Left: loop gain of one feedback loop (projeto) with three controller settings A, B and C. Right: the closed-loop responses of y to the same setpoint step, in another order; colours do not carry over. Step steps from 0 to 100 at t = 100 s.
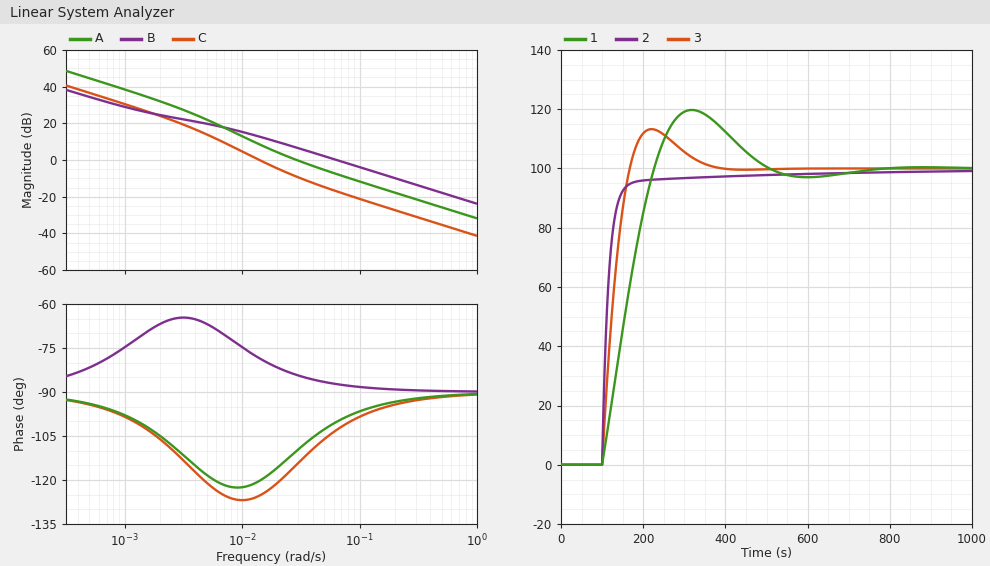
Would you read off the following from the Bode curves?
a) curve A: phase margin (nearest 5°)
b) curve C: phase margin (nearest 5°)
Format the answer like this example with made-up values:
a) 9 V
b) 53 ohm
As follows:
a) 70°
b) 55°
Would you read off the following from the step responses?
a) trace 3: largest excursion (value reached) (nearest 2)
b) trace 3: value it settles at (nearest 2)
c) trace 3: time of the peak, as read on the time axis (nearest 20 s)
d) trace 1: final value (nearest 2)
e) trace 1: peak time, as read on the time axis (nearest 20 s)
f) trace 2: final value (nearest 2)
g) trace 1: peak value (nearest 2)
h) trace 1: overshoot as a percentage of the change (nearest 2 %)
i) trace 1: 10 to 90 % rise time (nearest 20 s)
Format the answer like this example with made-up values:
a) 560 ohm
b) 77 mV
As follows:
a) 114
b) 100
c) 220 s
d) 100
e) 320 s
f) 100
g) 120
h) 20 %
i) 100 s
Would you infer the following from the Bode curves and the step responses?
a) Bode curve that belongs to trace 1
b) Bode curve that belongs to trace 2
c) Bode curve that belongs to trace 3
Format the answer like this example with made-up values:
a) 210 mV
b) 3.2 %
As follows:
a) C
b) B
c) A
